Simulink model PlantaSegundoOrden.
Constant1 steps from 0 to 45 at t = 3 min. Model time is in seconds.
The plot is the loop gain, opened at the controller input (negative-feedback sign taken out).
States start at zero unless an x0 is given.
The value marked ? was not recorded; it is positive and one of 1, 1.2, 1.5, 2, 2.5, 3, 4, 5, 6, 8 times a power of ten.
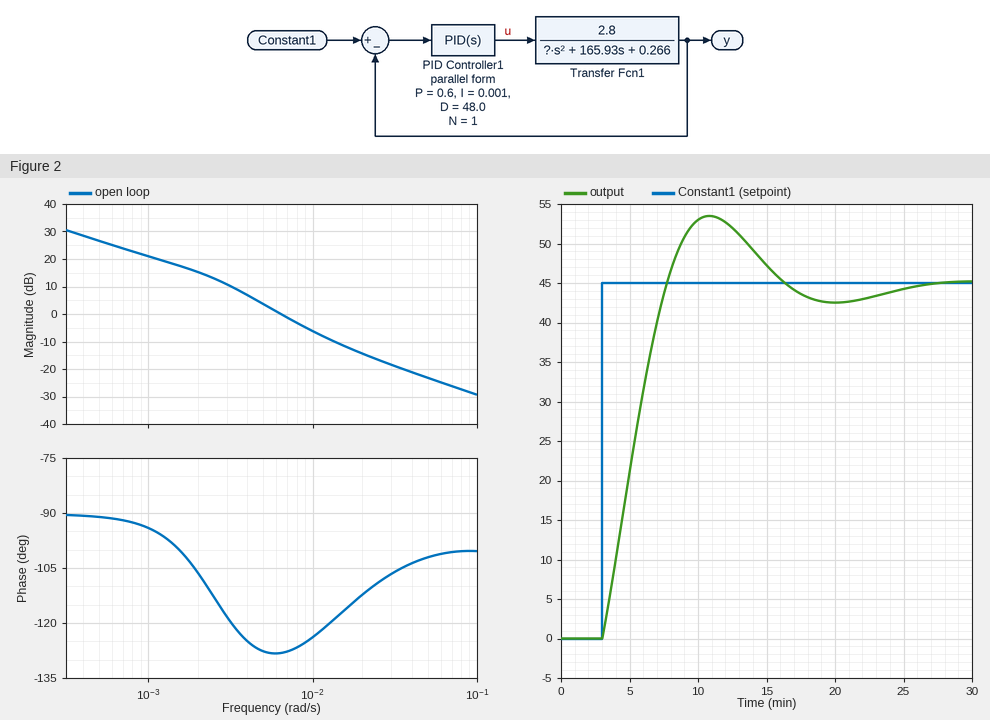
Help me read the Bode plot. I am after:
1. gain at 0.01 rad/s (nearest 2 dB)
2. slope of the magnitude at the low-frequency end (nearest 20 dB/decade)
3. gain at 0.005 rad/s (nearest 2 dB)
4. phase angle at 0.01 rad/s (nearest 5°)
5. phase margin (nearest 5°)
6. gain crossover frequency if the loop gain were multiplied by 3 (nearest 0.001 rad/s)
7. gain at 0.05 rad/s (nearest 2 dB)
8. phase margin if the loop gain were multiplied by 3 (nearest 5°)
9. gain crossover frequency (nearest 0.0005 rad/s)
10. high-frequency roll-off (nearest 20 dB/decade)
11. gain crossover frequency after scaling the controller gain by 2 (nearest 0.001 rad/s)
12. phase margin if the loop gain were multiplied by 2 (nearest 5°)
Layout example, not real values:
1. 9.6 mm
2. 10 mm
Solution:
1. -6 dB
2. -20 dB/decade
3. 4 dB
4. -125°
5. 50°
6. 0.013 rad/s
7. -24 dB
8. 60°
9. 0.0065 rad/s
10. -20 dB/decade
11. 0.010 rad/s
12. 55°
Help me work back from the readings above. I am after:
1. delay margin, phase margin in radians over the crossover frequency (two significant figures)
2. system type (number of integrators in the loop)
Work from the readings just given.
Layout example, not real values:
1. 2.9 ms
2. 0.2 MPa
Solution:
1. 130 s
2. 1
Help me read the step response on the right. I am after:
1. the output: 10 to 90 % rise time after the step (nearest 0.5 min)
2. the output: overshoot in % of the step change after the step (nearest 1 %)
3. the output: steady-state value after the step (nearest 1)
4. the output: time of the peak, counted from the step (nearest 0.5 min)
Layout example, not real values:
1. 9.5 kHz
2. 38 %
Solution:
1. 3.5 min
2. 19 %
3. 45
4. 8.0 min
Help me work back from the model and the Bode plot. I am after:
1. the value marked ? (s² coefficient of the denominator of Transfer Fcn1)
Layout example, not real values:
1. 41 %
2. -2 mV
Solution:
1. 40000
